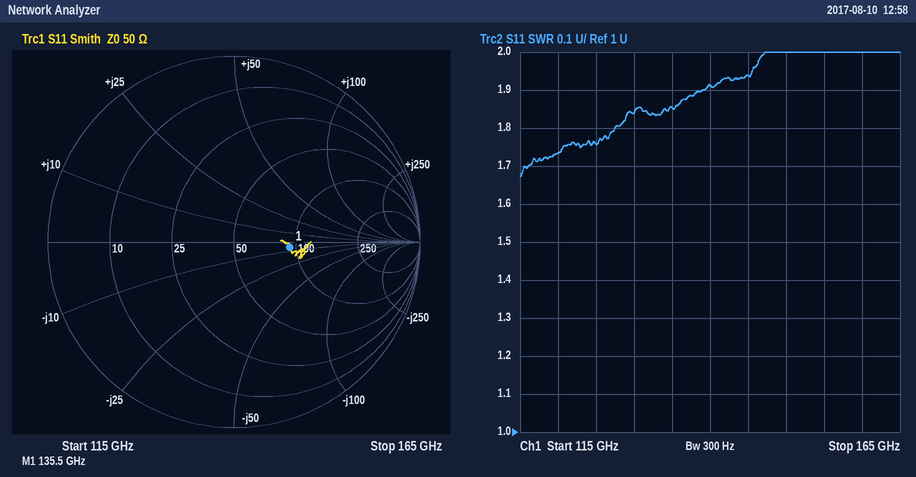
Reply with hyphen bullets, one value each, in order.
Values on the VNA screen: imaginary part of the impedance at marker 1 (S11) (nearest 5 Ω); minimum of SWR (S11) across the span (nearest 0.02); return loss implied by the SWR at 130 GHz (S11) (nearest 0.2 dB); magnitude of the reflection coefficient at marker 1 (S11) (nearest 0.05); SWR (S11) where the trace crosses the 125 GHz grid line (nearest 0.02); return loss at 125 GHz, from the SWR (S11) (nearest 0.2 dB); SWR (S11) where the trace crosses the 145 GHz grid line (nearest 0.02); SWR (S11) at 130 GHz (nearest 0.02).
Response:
- -5 Ω
- 1.68
- 10.6 dB
- 0.30
- 1.76
- 11.2 dB
- 1.94
- 1.84
